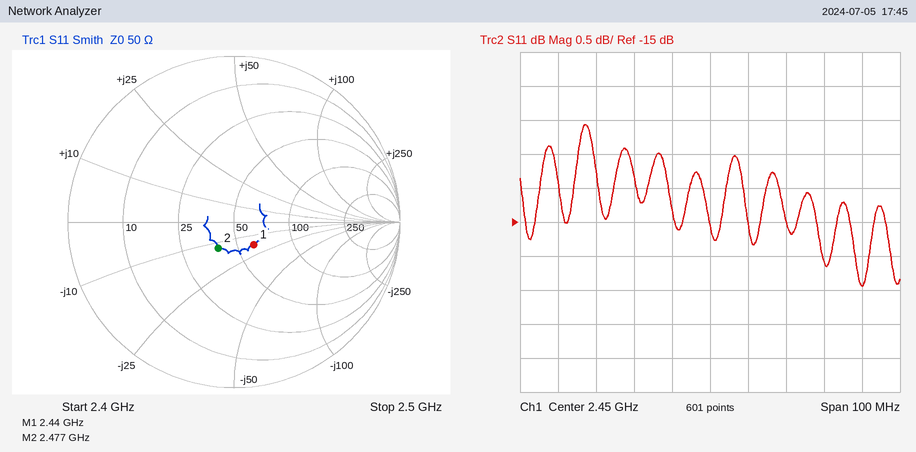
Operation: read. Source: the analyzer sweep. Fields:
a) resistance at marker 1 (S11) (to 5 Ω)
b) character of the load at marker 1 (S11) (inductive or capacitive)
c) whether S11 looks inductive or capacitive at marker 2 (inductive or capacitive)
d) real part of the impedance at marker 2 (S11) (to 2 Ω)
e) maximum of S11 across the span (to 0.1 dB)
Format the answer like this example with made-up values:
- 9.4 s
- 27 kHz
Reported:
- 60 Ω
- capacitive
- capacitive
- 40 Ω
- -13.6 dB
